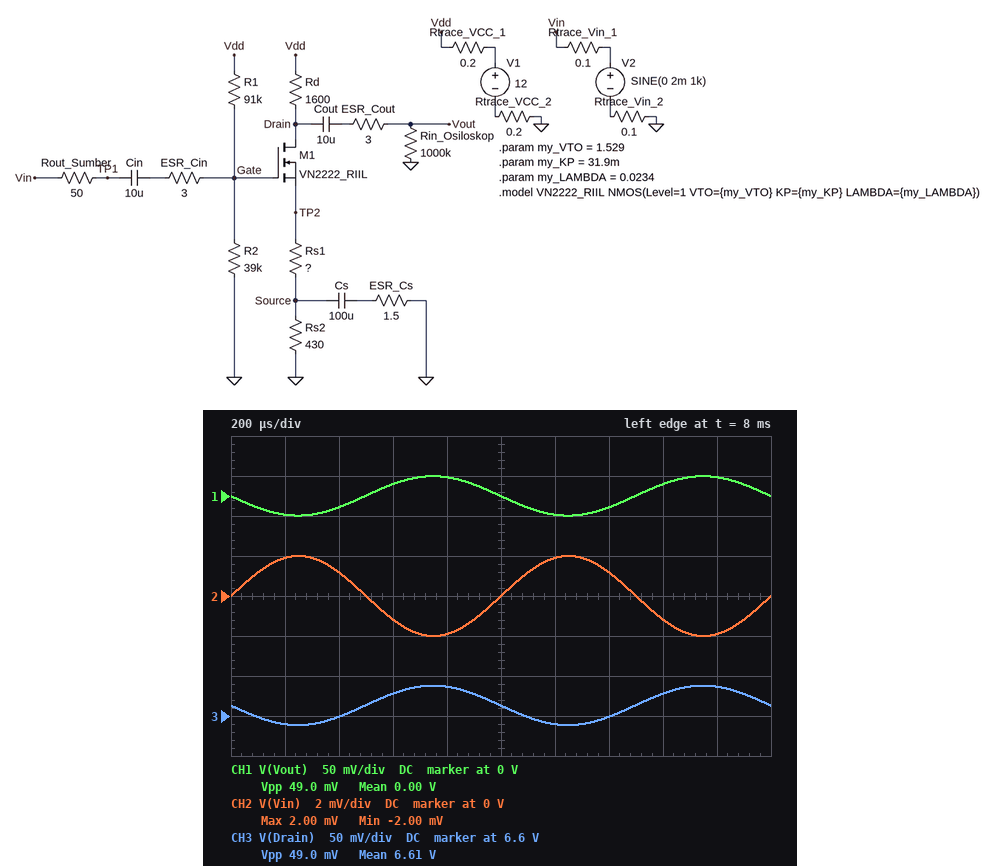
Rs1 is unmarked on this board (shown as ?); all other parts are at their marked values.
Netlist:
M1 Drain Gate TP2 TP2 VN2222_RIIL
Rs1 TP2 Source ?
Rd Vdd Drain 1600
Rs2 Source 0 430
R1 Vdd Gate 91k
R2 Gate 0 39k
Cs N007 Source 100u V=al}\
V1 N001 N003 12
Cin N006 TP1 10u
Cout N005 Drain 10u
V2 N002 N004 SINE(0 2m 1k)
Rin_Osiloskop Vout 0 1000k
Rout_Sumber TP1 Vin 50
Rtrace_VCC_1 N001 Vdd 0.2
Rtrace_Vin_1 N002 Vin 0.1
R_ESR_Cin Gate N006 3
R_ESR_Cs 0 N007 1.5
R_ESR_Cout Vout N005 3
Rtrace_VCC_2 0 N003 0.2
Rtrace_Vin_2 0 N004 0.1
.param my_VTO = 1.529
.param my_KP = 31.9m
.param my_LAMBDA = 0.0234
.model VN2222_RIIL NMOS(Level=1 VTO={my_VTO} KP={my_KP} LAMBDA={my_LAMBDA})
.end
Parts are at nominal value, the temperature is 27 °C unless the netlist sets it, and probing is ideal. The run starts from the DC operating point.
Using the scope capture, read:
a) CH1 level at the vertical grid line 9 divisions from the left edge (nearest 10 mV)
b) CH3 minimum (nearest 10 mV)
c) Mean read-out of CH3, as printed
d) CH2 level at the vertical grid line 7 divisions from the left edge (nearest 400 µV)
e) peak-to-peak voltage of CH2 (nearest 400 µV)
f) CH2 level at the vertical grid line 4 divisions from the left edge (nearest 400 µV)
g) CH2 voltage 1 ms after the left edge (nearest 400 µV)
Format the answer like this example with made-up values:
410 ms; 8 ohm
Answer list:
20 mV; 6.59 V; 6.61 V; 1.2 mV; 4.0 mV; -2.0 mV; 0 V
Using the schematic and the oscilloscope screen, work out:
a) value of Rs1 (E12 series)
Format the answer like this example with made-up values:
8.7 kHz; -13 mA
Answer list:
56 Ω
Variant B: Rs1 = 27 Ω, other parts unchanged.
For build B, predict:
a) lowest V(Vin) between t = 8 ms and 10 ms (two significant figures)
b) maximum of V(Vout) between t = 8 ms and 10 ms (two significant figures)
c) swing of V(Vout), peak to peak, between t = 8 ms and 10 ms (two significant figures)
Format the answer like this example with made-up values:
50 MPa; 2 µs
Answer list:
-2.0 mV; 32 mV; 64 mV
